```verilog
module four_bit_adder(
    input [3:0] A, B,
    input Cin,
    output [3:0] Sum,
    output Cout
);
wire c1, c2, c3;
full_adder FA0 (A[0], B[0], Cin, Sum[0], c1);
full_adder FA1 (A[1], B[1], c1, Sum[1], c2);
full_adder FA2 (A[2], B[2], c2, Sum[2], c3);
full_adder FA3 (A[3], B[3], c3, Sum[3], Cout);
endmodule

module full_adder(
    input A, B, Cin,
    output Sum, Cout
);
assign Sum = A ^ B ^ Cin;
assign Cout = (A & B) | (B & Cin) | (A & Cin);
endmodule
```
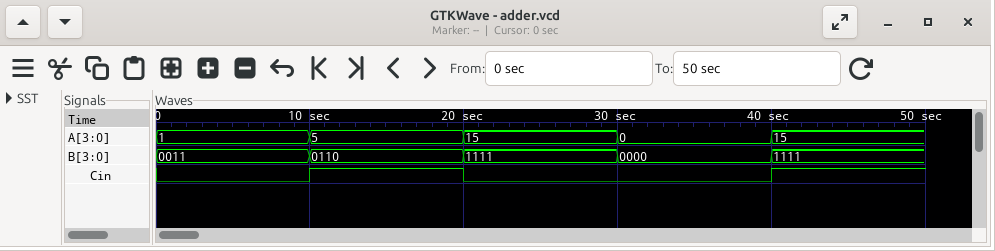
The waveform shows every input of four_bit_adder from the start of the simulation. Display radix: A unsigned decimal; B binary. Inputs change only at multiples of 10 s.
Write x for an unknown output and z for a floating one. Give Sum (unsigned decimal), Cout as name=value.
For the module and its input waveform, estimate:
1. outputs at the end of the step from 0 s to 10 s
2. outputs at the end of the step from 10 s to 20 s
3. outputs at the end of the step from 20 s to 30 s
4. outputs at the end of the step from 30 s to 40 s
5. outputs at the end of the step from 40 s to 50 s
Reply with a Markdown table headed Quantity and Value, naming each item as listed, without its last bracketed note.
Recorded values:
| Quantity | Value |
|---|---|
| outputs at the end of the step from 0 s to 10 s | Sum=4, Cout=0 |
| outputs at the end of the step from 10 s to 20 s | Sum=12, Cout=0 |
| outputs at the end of the step from 20 s to 30 s | Sum=14, Cout=1 |
| outputs at the end of the step from 30 s to 40 s | Sum=0, Cout=0 |
| outputs at the end of the step from 40 s to 50 s | Sum=15, Cout=1 |
